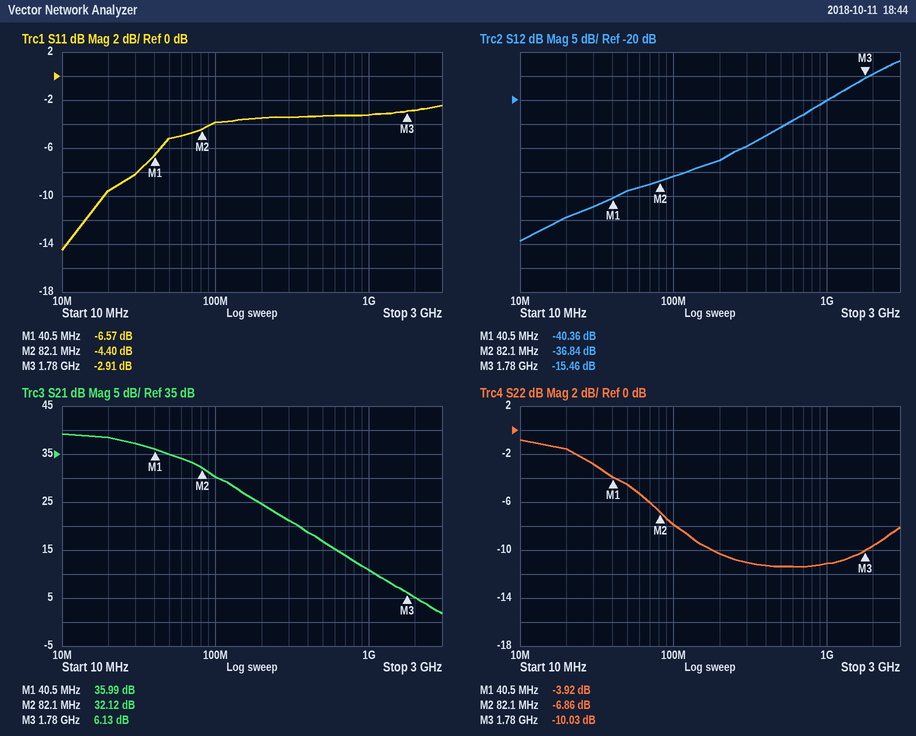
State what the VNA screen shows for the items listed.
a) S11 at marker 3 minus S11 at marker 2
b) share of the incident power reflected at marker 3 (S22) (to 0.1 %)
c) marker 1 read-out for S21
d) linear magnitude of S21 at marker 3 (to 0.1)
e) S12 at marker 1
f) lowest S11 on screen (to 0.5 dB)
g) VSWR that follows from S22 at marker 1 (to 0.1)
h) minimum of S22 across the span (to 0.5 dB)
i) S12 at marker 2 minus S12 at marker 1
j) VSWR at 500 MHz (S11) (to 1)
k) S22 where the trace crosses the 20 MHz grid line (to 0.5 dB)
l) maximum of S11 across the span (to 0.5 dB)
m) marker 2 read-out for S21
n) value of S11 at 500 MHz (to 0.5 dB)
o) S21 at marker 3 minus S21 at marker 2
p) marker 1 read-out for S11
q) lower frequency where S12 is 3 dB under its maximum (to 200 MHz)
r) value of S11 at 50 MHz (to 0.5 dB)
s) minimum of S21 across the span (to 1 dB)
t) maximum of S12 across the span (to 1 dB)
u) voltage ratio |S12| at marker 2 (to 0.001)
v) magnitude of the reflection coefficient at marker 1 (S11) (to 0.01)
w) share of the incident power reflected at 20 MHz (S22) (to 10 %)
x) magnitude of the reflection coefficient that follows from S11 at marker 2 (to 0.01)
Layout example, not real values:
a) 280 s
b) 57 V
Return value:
a) 1.49 dB
b) 9.9 %
c) 35.99 dB
d) 2.0
e) -40.36 dB
f) -14.5 dB
g) 4.5
h) -11.5 dB
i) 3.52 dB
j) 5
k) -1.5 dB
l) -2.5 dB
m) 32.12 dB
n) -3.5 dB
o) -25.99 dB
p) -6.57 dB
q) 2.0 GHz
r) -5.0 dB
s) 2 dB
t) -12 dB
u) 0.014
v) 0.47
w) 70 %
x) 0.60
